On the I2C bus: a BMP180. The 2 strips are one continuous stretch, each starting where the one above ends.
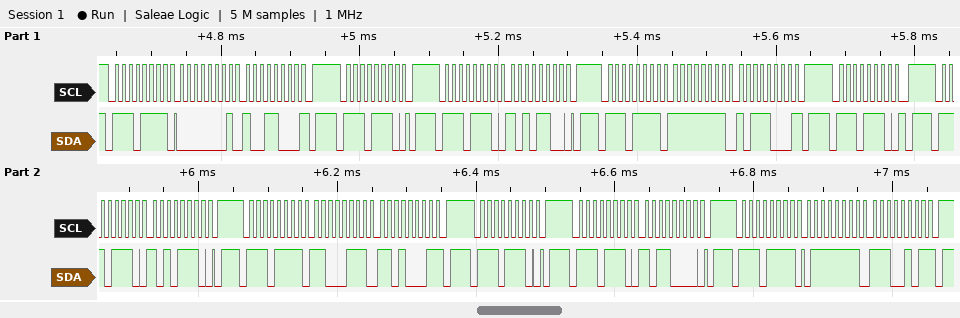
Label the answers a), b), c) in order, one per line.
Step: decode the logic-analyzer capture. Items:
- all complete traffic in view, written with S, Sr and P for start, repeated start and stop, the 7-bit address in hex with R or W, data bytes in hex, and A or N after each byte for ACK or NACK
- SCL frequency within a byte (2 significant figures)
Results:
a) S 77R A 01 A 98 N P S 77W A P S 77W A AC A P S 77R A FF A B8 N P S 77W A P S 77W A AE A P S 77R A C7 A D1 N P S 77W A P S 77W A B0 A P S 77R A 7F A E5 N P
b) 100 kHz
